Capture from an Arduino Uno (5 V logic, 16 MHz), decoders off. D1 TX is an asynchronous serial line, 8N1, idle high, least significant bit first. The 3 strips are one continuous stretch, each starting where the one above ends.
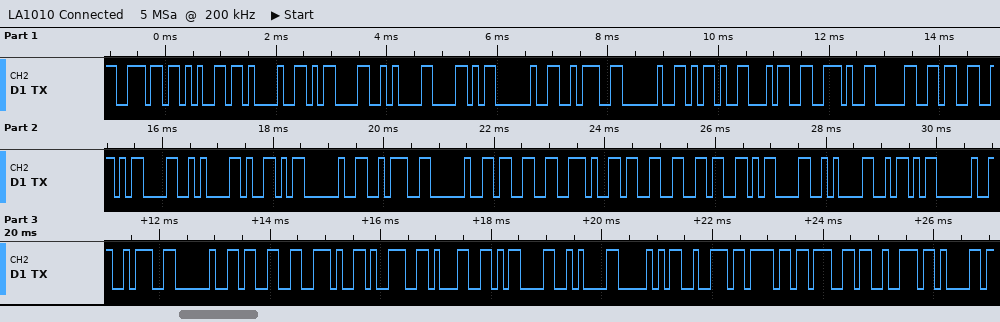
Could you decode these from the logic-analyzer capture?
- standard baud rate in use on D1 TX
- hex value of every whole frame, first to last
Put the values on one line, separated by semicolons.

9600 baud; 6E 65 21 0D 0A 58 20 3A 20 2D 34 2E 30 33 0D 0A 59 20 3A 20 33 2E 33 36 0D 0A 5A 20 3A 20 33 2E 39 31 0D 0A 50 72 6F 67 72 61
